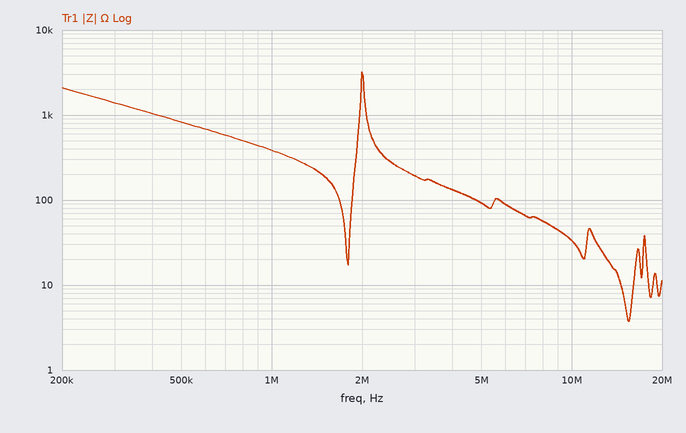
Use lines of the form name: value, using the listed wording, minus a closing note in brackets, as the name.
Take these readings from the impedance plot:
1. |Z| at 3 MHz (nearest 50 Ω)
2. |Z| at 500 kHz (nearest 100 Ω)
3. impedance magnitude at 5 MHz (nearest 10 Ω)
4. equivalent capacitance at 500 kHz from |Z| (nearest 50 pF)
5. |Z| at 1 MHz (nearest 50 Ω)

|Z| at 3 MHz: 200 Ω
|Z| at 500 kHz: 800 Ω
impedance magnitude at 5 MHz: 90 Ω
equivalent capacitance at 500 kHz from |Z|: 400 pF
|Z| at 1 MHz: 400 Ω
